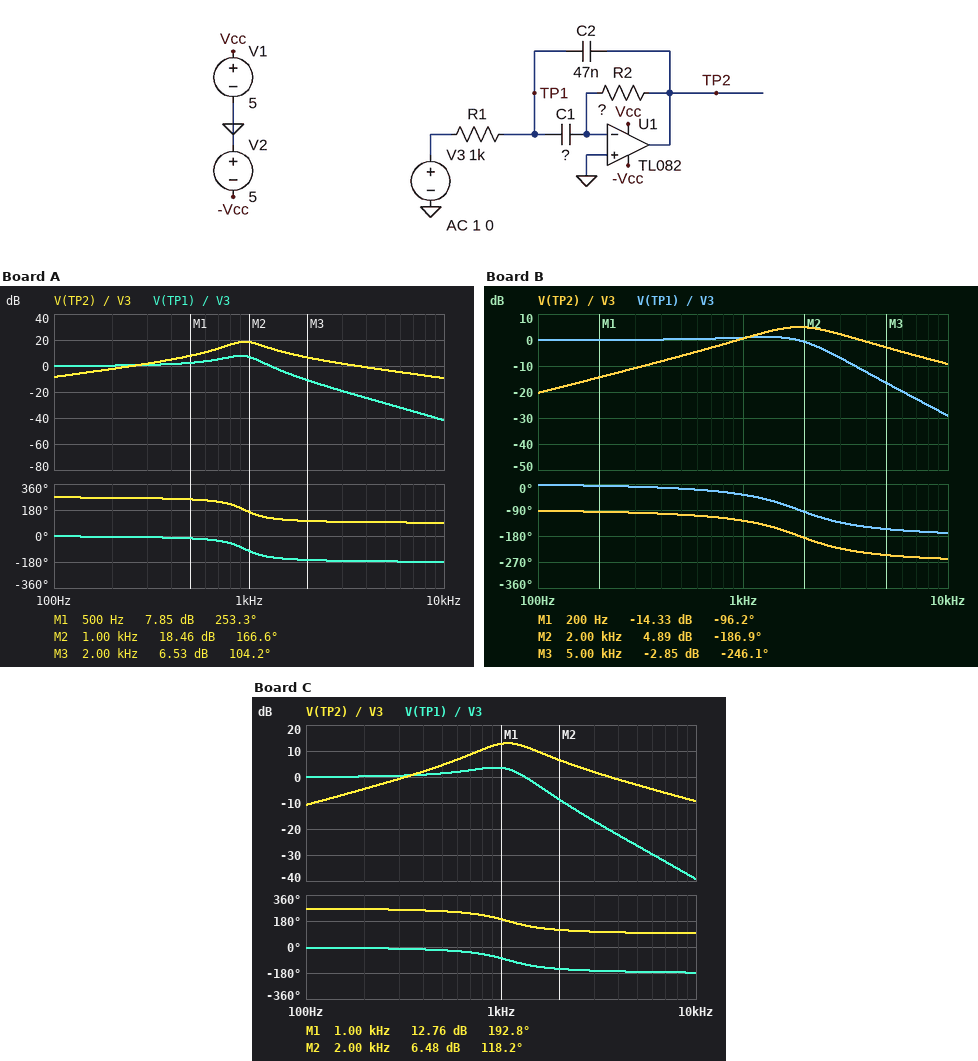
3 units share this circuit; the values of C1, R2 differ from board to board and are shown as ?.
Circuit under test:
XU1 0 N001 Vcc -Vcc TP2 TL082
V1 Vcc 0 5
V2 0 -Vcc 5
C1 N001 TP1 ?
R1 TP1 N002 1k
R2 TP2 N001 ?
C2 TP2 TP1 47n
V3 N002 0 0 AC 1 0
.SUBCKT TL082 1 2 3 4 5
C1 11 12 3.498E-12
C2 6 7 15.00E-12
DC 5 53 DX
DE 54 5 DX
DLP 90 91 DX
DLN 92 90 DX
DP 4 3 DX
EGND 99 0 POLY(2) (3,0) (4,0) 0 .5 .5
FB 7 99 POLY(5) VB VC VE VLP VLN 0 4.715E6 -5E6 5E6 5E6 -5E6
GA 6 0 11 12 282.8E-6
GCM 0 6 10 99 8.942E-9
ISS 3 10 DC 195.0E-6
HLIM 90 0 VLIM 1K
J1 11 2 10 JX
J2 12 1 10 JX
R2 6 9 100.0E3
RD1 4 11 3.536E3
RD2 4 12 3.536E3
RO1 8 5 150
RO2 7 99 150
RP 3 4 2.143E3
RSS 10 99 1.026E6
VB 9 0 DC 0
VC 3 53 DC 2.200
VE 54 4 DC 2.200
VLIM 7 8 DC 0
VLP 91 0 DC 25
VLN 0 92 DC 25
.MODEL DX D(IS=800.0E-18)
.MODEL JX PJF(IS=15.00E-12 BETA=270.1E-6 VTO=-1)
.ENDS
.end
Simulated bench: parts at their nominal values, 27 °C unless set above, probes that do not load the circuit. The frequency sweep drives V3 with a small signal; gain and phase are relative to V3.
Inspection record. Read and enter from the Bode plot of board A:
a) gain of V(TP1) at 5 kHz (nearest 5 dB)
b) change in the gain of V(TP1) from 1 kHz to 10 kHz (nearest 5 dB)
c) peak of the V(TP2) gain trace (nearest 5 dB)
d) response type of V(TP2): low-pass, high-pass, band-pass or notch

-30 dB
-50 dB
20 dB
band-pass
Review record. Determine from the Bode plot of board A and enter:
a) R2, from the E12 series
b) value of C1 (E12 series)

27 kΩ
22 nF
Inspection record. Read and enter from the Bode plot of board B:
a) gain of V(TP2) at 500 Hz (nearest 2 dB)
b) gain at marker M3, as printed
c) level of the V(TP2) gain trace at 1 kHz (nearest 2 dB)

-6 dB
-2.85 dB
0 dB
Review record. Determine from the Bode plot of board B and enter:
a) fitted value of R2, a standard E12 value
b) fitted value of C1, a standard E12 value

3.9 kΩ
39 nF
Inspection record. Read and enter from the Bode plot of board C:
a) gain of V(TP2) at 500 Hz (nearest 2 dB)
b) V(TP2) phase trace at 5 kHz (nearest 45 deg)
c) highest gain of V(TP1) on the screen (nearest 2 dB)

4 dB
90 deg
4 dB
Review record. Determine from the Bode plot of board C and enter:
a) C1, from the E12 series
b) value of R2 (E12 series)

56 nF
8.2 kΩ
